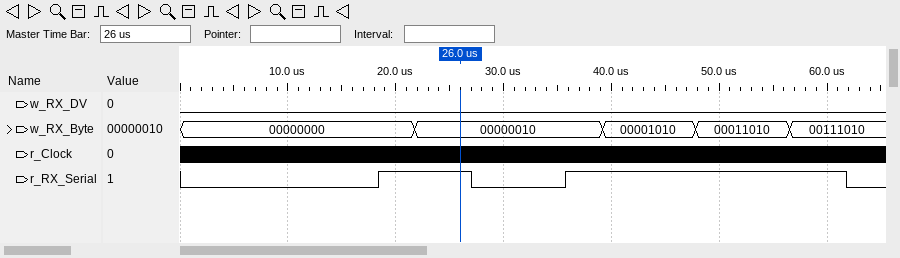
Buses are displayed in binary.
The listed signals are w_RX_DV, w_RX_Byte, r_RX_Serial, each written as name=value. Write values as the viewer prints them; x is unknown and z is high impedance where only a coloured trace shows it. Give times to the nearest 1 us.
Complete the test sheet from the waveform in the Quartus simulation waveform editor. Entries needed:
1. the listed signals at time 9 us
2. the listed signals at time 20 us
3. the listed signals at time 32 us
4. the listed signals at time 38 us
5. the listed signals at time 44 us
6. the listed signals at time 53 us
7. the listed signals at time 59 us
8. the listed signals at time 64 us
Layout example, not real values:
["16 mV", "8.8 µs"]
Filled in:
["w_RX_DV=0, w_RX_Byte=00000000, r_RX_Serial=0", "w_RX_DV=0, w_RX_Byte=00000000, r_RX_Serial=1", "w_RX_DV=0, w_RX_Byte=00000010, r_RX_Serial=0", "w_RX_DV=0, w_RX_Byte=00000010, r_RX_Serial=1", "w_RX_DV=0, w_RX_Byte=00001010, r_RX_Serial=1", "w_RX_DV=0, w_RX_Byte=00011010, r_RX_Serial=1", "w_RX_DV=0, w_RX_Byte=00111010, r_RX_Serial=1", "w_RX_DV=0, w_RX_Byte=00111010, r_RX_Serial=0"]
